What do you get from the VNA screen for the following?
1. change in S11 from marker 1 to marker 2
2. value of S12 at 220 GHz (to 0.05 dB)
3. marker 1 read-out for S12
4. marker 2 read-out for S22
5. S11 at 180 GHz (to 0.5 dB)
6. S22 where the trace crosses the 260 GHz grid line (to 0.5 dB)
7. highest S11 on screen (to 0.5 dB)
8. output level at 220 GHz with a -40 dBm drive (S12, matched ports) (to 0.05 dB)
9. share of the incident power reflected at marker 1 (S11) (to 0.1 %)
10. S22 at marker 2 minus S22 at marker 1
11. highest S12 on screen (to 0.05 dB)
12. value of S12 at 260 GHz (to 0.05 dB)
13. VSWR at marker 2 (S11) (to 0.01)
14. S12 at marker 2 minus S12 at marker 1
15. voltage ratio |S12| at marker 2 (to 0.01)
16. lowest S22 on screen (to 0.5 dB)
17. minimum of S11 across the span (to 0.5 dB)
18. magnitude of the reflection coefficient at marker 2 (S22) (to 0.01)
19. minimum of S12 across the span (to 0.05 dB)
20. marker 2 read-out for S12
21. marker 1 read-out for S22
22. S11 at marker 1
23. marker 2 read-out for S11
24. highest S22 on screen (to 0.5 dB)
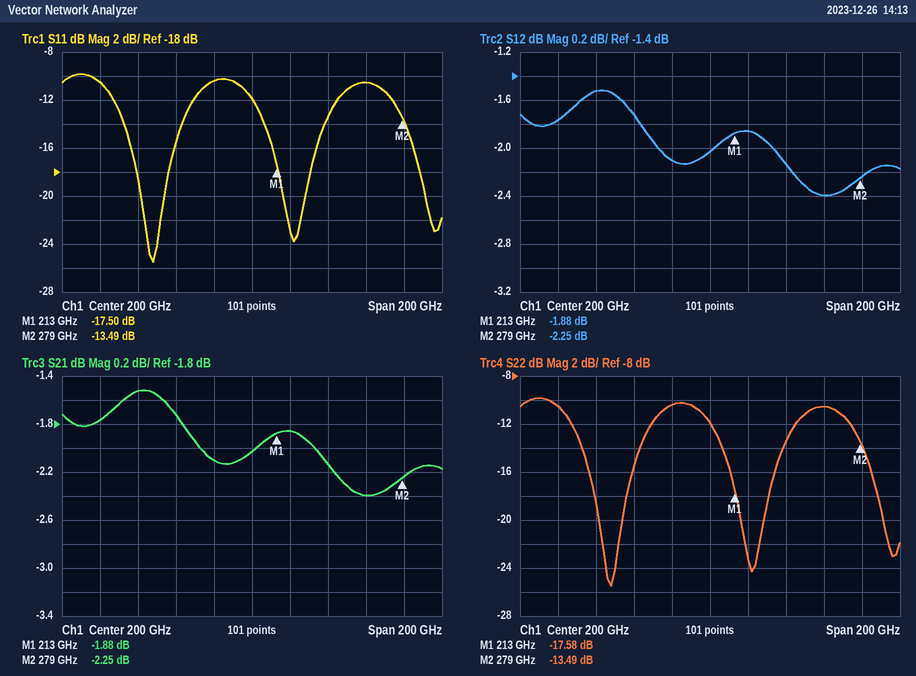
4.01 dB
-1.85 dB
-1.88 dB
-13.49 dB
-10.5 dB
-10.5 dB
-10.0 dB
-41.85 dBm
1.8 %
4.09 dB
-1.50 dB
-2.40 dB
1.54
-0.37 dB
0.77
-25.5 dB
-25.5 dB
0.21
-2.40 dB
-2.25 dB
-17.58 dB
-17.50 dB
-13.49 dB
-10.0 dB
